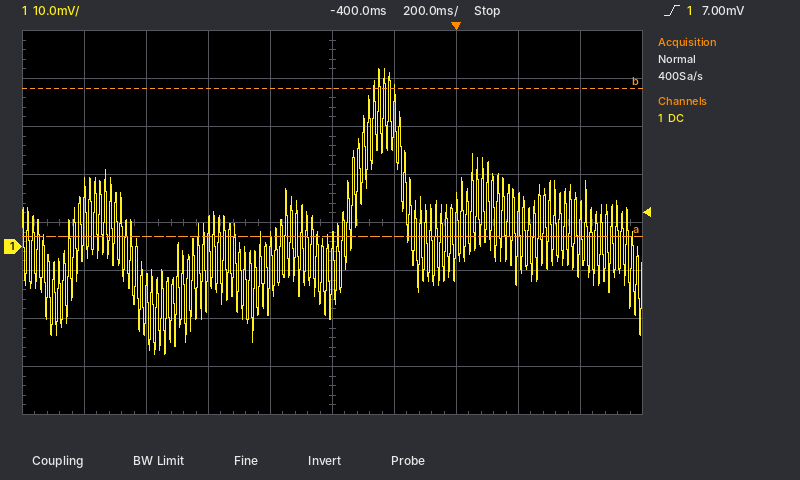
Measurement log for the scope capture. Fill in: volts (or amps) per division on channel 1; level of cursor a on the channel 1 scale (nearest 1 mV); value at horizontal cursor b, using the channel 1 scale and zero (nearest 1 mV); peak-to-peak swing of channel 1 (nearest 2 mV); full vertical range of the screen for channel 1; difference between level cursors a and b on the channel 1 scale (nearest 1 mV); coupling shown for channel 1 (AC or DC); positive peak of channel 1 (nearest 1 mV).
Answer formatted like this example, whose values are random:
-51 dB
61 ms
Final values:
10 mV
2 mV
33 mV
60 mV
80 mV
31 mV
DC
37 mV
